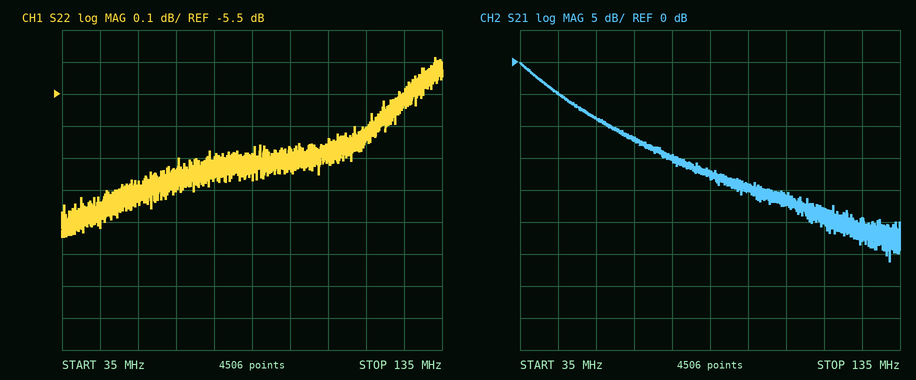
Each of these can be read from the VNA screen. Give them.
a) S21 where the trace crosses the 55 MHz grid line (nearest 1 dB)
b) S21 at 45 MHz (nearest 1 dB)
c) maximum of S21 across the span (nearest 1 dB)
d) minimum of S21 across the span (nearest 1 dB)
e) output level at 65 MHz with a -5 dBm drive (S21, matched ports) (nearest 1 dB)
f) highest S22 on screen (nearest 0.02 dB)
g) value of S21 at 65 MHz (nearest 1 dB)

-9 dB
-5 dB
0 dB
-31 dB
-17 dBm
-5.38 dB
-12 dB
